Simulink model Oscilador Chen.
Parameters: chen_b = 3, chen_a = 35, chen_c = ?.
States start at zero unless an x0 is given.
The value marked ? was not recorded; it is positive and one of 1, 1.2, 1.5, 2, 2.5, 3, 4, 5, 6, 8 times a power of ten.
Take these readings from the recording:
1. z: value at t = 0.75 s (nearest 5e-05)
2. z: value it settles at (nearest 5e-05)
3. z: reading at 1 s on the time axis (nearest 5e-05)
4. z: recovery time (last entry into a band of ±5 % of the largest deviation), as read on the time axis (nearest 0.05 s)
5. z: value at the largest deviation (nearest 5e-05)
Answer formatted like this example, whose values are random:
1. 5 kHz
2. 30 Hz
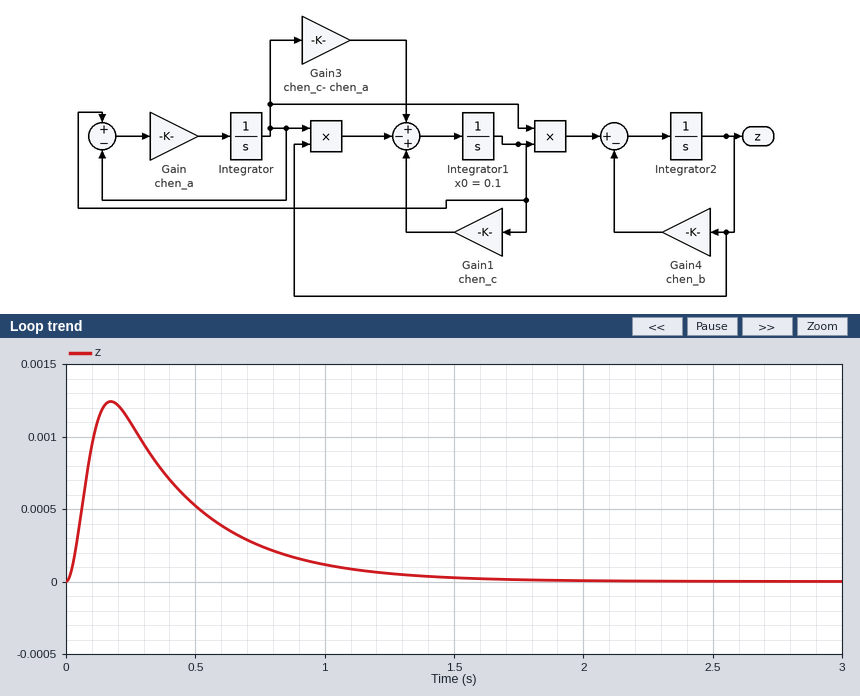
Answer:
1. 0.00025
2. 0.00000
3. 0.00010
4. 1.20 s
5. 0.00125
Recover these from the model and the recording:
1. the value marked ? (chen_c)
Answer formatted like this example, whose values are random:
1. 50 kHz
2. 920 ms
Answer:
1. 15
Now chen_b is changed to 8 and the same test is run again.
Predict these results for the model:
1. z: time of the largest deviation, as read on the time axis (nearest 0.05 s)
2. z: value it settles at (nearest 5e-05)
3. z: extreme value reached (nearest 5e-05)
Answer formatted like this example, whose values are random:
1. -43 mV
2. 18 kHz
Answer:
1. 0.15 s
2. 0.00000
3. 0.00090
